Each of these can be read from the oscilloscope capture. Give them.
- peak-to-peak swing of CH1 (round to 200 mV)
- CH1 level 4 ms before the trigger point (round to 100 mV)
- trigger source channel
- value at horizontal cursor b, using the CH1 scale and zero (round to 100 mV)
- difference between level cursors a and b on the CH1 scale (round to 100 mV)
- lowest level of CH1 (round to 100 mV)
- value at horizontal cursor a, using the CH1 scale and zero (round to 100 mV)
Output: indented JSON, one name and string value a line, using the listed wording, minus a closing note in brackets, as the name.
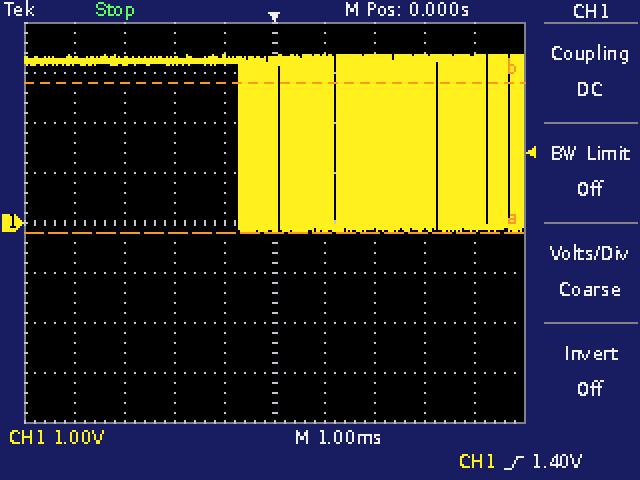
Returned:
{
  "peak-to-peak swing of CH1": "3.6 V",
  "CH1 level 4 ms before the trigger point": "3.2 V",
  "trigger source channel": "CH1",
  "value at horizontal cursor b, using the CH1 scale and zero": "2.8 V",
  "difference between level cursors a and b on the CH1 scale": "3.0 V",
  "lowest level of CH1": "-200 mV",
  "value at horizontal cursor a, using the CH1 scale and zero": "-200 mV"
}
